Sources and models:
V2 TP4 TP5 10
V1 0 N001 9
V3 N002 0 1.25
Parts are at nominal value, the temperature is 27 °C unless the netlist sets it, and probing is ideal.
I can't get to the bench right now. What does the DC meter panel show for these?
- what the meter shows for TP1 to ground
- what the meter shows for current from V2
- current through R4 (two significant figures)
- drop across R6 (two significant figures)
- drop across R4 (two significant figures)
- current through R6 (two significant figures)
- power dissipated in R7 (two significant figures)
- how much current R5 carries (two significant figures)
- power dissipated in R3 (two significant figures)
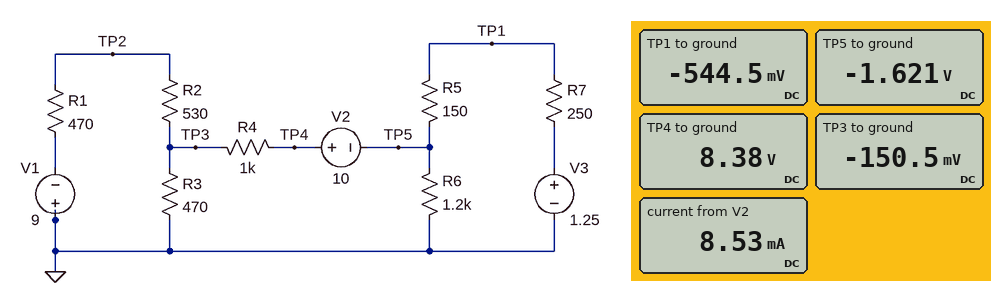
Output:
-544.5 mV
8.53 mA
8.5 mA
1.6 V
8.5 V
1.4 mA
13 mW
7.2 mA
48 µW
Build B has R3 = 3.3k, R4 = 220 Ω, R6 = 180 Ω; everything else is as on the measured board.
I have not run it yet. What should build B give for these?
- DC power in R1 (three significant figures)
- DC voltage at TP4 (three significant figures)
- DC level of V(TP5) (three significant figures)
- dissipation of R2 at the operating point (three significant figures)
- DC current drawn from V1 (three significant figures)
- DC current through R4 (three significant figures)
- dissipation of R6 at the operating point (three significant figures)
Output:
92.6 mW
8.46 V
-1.54 V
104 mW
14.0 mA
15.6 mA
13.2 mW
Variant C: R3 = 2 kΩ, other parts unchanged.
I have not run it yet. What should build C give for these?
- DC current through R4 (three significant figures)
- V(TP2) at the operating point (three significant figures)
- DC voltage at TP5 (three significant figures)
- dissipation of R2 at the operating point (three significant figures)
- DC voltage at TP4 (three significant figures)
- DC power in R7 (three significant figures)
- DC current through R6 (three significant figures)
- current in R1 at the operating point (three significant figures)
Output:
8.61 mA
-4.89 V
-1.65 V
40.5 mW
8.35 V
13.1 mW
1.37 mA
8.74 mA
